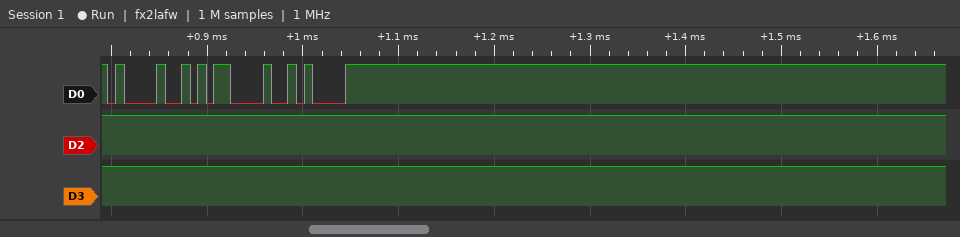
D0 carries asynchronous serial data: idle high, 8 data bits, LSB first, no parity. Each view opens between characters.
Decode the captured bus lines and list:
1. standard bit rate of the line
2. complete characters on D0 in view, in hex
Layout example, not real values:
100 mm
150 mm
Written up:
115200 baud
21, 0D, 0A
